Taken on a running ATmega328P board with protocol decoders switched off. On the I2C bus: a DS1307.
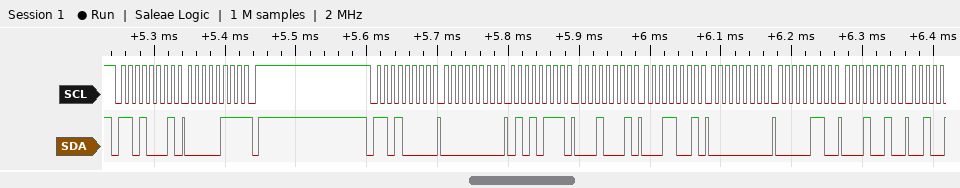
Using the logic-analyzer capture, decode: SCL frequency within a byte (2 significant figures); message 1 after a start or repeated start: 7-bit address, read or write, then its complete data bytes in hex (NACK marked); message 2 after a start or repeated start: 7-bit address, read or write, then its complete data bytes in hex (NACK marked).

100 kHz
0x68 read: 07 NACK
0x68 write: 00 57 11 19 00 06 12
